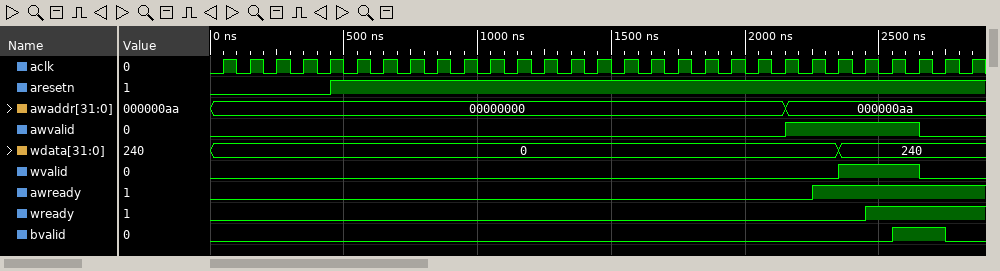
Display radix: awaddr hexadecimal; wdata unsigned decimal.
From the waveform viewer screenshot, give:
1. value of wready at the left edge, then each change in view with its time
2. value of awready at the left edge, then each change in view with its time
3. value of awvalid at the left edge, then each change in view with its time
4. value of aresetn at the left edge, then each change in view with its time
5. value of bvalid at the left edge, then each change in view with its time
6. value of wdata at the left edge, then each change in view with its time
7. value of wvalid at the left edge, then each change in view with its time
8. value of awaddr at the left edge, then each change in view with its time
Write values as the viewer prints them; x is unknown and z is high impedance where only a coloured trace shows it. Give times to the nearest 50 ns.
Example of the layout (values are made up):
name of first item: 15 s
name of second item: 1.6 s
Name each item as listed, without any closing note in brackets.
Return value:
value of wready at the left edge, then each change in view with its time: 0, 1 at 2450 ns
value of awready at the left edge, then each change in view with its time: 0, 1 at 2250 ns
value of awvalid at the left edge, then each change in view with its time: 0, 1 at 2150 ns, 0 at 2650 ns
value of aresetn at the left edge, then each change in view with its time: 0, 1 at 450 ns
value of bvalid at the left edge, then each change in view with its time: 0, 1 at 2550 ns, 0 at 2750 ns
value of wdata at the left edge, then each change in view with its time: 0, 240 at 2350 ns
value of wvalid at the left edge, then each change in view with its time: 0, 1 at 2350 ns, 0 at 2650 ns
value of awaddr at the left edge, then each change in view with its time: 00000000, 000000aa at 2150 ns
